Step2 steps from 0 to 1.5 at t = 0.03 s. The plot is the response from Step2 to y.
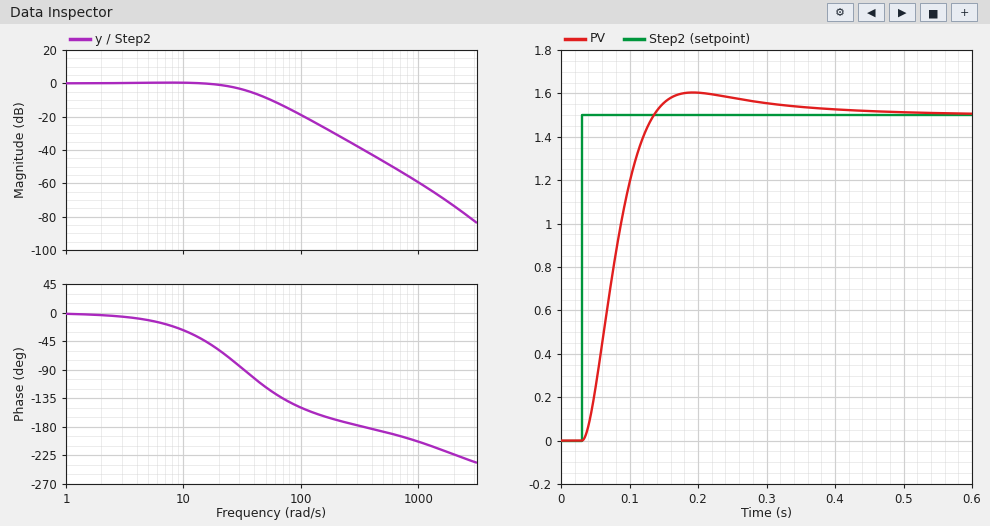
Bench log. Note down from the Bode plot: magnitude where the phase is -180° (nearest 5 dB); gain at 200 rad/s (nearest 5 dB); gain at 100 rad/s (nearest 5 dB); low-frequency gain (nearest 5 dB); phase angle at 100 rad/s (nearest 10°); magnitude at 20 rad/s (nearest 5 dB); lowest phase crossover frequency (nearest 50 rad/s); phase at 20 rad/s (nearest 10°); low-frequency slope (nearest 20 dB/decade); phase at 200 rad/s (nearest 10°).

-40 dB
-30 dB
-20 dB
0 dB
-150°
0 dB
350 rad/s
-60°
0 dB/decade
-170°
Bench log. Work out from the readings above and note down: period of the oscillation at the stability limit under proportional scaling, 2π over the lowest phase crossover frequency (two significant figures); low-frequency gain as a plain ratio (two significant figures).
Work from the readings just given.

0.018 s
1.0
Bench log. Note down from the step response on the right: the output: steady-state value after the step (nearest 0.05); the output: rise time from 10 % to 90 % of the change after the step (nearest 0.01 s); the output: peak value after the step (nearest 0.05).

1.50
0.07 s
1.60
